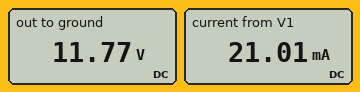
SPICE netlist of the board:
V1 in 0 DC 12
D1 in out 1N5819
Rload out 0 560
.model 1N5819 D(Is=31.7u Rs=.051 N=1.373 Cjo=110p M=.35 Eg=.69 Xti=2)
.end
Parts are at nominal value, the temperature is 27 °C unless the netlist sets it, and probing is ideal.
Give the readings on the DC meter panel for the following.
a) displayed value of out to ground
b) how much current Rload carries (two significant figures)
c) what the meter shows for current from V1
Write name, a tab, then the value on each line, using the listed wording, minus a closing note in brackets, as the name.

displayed value of out to ground	11.77 V
how much current Rload carries	21 mA
what the meter shows for current from V1	21.01 mA
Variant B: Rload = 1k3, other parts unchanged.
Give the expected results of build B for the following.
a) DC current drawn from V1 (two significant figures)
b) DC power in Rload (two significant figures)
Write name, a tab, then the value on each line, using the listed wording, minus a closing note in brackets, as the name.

DC current drawn from V1	9.1 mA
DC power in Rload	110 mW
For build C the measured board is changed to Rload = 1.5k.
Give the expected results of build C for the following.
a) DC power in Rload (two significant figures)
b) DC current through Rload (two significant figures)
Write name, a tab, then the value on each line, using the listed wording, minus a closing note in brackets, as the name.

DC power in Rload	93 mW
DC current through Rload	7.9 mA
